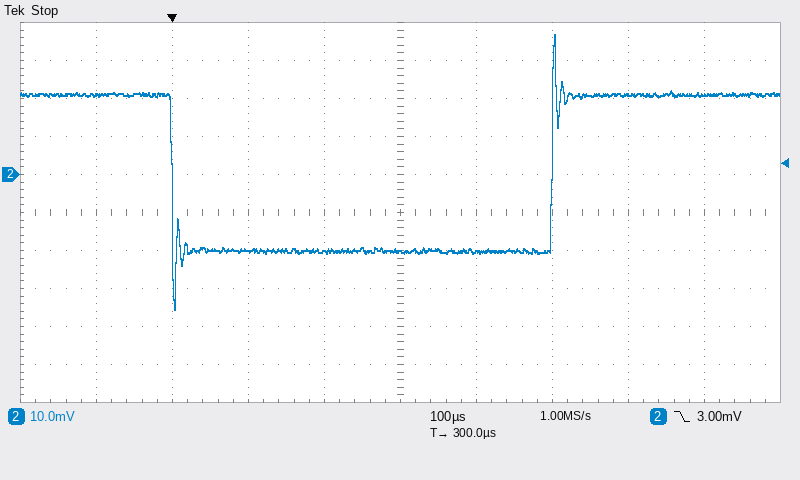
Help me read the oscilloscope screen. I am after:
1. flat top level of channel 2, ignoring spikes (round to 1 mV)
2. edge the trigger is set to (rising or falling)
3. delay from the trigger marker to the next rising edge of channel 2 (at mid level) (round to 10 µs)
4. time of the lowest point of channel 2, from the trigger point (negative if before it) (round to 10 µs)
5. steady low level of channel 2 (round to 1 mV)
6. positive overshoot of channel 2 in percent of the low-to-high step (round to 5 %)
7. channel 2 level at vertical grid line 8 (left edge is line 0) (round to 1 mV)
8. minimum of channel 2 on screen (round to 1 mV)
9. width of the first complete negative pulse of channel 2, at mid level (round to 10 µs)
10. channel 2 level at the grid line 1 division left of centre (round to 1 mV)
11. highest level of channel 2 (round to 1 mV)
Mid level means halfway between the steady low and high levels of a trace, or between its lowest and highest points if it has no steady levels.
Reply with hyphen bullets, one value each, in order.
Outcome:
- 21 mV
- falling
- 500 µs
- 0 µs
- -20 mV
- 40 %
- 21 mV
- -36 mV
- 500 µs
- -20 mV
- 37 mV
